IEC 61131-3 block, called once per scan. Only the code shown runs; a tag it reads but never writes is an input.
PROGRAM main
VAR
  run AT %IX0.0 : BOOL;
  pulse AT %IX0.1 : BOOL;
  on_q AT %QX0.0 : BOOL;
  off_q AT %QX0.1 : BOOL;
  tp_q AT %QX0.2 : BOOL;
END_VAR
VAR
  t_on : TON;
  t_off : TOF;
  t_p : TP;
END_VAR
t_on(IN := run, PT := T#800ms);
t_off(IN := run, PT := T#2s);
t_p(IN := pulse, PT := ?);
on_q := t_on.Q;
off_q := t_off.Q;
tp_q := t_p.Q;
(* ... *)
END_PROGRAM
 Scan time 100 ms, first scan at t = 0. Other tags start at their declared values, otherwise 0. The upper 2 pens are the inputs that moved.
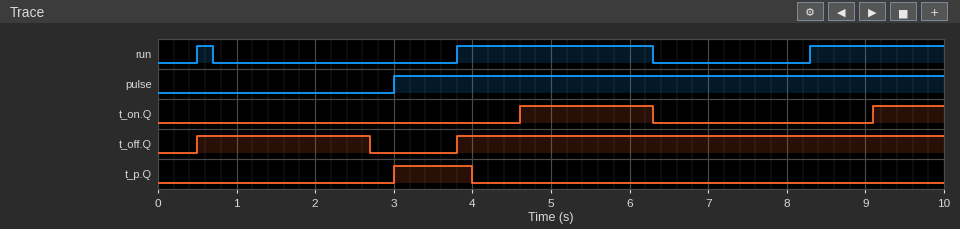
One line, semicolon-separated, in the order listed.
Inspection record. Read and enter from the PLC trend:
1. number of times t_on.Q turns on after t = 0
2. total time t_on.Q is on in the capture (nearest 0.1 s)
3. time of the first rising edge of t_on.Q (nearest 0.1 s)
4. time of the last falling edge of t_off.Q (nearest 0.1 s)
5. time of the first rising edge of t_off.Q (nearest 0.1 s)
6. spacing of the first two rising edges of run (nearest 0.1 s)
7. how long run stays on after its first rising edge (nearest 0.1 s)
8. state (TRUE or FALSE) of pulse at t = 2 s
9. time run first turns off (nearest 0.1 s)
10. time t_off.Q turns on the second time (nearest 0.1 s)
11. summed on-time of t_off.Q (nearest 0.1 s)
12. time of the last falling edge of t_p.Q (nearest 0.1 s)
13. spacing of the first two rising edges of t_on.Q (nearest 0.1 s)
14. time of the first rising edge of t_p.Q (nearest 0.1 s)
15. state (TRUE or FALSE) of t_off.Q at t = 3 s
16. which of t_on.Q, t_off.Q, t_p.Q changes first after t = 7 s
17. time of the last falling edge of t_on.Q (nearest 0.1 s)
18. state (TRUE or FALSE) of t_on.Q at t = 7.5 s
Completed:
2; 2.6 s; 4.6 s; 2.7 s; 0.5 s; 3.3 s; 0.2 s; FALSE; 0.7 s; 3.8 s; 8.4 s; 4.0 s; 4.5 s; 3.0 s; FALSE; t_on.Q; 6.3 s; FALSE
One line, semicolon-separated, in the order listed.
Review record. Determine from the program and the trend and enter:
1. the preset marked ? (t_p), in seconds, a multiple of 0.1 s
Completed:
1.0 s
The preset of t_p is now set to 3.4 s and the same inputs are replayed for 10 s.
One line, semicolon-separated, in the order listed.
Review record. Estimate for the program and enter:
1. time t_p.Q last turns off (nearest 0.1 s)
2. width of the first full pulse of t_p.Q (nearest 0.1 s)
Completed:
6.4 s; 3.4 s
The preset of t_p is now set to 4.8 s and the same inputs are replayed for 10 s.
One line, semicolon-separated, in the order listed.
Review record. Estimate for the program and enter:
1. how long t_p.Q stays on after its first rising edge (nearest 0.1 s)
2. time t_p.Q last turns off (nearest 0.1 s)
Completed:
4.8 s; 7.8 s
